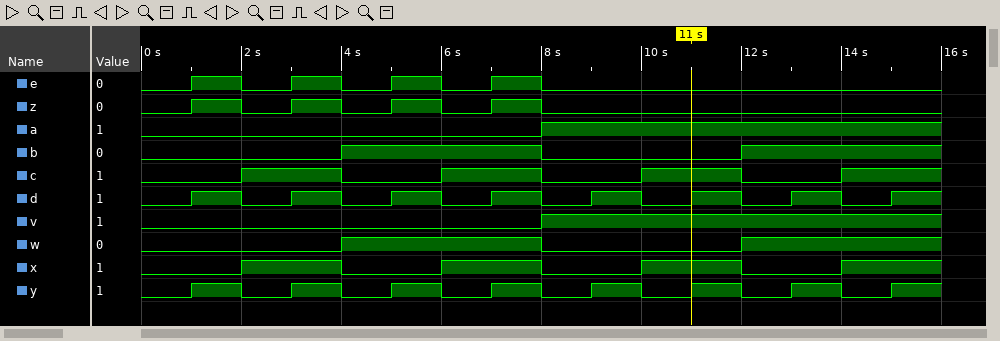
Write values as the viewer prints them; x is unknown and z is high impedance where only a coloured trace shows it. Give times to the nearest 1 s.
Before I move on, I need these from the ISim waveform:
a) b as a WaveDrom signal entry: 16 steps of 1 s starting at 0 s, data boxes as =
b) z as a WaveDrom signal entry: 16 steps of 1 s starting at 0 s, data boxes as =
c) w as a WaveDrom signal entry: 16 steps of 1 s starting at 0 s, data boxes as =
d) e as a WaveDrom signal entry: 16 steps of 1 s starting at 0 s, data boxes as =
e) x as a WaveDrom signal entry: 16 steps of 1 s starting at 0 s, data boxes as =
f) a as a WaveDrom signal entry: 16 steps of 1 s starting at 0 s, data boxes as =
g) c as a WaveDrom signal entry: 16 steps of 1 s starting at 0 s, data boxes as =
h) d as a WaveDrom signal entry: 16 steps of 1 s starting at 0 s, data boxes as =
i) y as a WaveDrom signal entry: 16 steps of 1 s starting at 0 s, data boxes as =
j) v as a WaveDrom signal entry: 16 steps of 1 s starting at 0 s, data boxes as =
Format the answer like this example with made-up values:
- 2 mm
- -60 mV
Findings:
- {name: 'b', wave: '0...1...0...1...'}
- {name: 'z', wave: '010101010.......'}
- {name: 'w', wave: '0...1...0...1...'}
- {name: 'e', wave: '010101010.......'}
- {name: 'x', wave: '0.1.0.1.0.1.0.1.'}
- {name: 'a', wave: '0.......1.......'}
- {name: 'c', wave: '0.1.0.1.0.1.0.1.'}
- {name: 'd', wave: '0101010101010101'}
- {name: 'y', wave: '0101010101010101'}
- {name: 'v', wave: '0.......1.......'}
